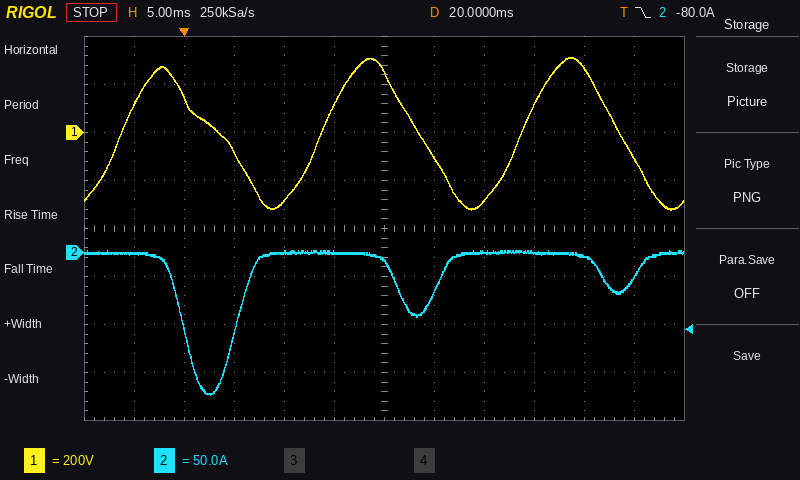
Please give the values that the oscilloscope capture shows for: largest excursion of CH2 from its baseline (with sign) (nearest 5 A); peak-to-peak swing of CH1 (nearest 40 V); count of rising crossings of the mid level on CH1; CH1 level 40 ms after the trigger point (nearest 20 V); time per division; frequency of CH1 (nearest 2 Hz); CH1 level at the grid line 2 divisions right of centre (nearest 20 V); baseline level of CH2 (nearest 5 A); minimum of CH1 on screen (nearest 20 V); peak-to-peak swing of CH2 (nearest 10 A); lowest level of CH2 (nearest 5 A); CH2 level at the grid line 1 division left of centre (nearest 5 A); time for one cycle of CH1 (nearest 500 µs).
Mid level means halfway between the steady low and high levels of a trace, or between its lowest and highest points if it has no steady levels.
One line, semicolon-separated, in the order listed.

-150 A; 640 V; 3; 260 V; 5 ms; 50 Hz; -280 V; 0 A; -320 V; 150 A; -150 A; 0 A; 20.0 ms
